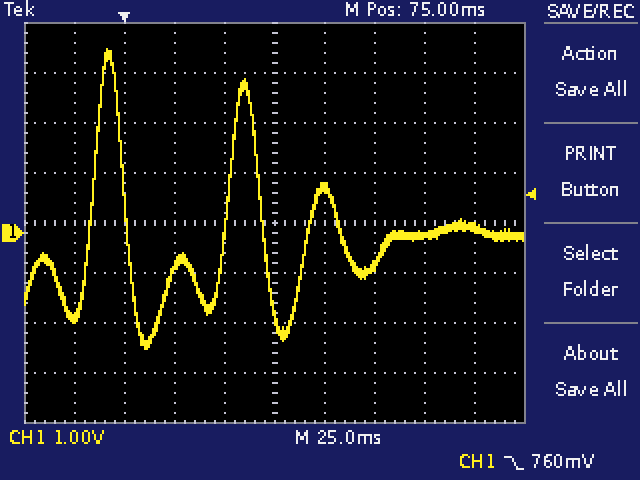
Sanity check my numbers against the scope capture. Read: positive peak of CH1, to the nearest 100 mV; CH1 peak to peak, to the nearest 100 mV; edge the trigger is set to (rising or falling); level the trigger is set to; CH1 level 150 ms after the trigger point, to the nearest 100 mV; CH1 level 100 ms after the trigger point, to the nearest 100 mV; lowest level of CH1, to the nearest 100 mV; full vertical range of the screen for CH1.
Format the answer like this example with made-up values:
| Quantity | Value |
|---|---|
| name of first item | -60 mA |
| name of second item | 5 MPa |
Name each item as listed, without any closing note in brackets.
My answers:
| Quantity | Value |
|---|---|
| positive peak of CH1, to the nearest 100 mV | 3.7 V |
| CH1 peak to peak, to the nearest 100 mV | 6.0 V |
| edge the trigger is set to | falling |
| level the trigger is set to | 760 mV |
| CH1 level 150 ms after the trigger point, to the nearest 100 mV | -100 mV |
| CH1 level 100 ms after the trigger point, to the nearest 100 mV | 900 mV |
| lowest level of CH1, to the nearest 100 mV | -2.3 V |
| full vertical range of the screen for CH1 | 8 V |
